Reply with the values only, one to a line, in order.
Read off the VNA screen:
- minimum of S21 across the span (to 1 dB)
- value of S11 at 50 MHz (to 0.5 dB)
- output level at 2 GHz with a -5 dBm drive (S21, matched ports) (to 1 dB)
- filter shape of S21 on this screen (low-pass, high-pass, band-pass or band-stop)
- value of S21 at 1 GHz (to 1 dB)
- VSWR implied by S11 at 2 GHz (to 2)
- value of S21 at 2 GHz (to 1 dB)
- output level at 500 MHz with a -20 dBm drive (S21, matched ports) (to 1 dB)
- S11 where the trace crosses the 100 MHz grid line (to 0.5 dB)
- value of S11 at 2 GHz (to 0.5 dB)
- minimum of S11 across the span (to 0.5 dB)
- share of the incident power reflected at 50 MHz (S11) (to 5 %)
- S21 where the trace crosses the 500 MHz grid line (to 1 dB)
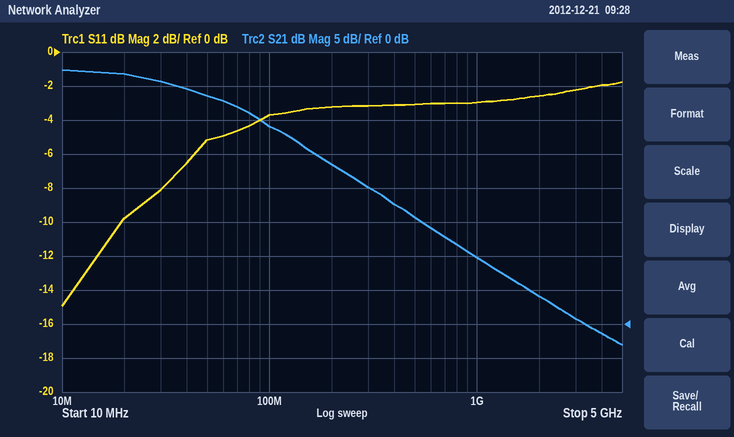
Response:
-3 dB
-5.0 dB
-1 dBm
low-pass
10 dB
6
4 dB
-4 dBm
-3.5 dB
-2.5 dB
-15.0 dB
30 %
16 dB
